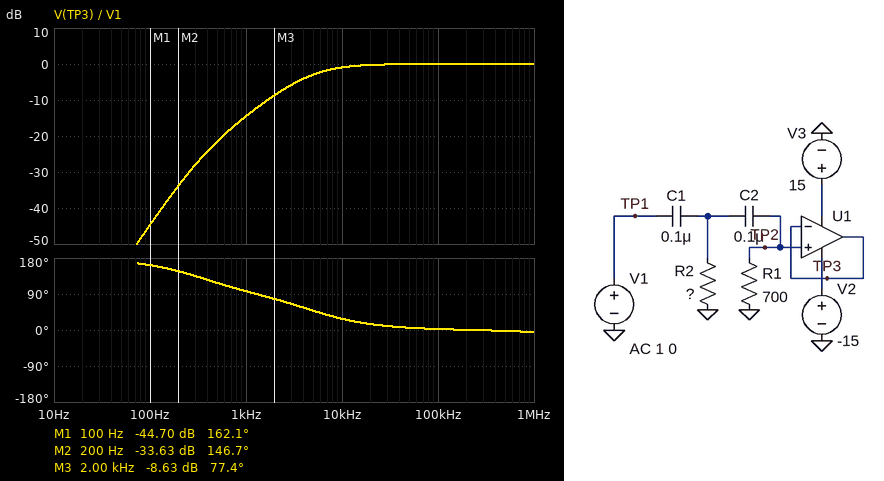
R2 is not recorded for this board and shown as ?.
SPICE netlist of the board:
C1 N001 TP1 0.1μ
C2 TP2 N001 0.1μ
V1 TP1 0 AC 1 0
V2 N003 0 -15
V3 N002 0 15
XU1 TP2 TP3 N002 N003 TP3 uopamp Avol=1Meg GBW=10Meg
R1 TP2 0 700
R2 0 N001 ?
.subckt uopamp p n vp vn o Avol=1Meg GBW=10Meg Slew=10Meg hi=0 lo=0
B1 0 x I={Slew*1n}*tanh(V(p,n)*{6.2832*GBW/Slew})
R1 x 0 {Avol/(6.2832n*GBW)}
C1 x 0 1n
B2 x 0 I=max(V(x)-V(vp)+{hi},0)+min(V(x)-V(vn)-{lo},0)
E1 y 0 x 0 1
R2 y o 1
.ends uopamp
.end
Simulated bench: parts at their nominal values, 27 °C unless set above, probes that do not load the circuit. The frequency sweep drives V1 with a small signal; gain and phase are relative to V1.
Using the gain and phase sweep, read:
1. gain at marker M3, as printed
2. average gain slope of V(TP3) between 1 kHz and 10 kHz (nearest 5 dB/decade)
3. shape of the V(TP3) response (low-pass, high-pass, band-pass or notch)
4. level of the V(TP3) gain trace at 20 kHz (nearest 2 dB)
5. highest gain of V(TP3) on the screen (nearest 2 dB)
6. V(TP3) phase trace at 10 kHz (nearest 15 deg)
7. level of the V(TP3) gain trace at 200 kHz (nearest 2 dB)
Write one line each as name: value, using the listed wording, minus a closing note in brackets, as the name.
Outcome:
gain at marker M3, as printed: -8.63 dB
average gain slope of V(TP3) between 1 kHz and 10 kHz: 15 dB/decade
shape of the V(TP3) response: high-pass
level of the V(TP3) gain trace at 20 kHz: 0 dB
highest gain of V(TP3) on the screen: 0 dB
V(TP3) phase trace at 10 kHz: 30 deg
level of the V(TP3) gain trace at 200 kHz: 0 dB
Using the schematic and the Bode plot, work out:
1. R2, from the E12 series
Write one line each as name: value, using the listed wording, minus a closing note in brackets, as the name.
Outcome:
R2, from the E12 series: 2.2 kΩ
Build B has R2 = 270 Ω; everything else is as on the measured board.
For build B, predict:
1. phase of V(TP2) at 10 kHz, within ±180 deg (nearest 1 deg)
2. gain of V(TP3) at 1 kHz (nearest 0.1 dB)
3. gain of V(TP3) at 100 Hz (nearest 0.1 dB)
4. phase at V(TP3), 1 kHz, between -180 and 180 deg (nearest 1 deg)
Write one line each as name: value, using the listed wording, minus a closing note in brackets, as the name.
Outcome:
phase of V(TP2) at 10 kHz, within ±180 deg: 50 deg
gain of V(TP3) at 1 kHz: -24.2 dB
gain of V(TP3) at 100 Hz: -62.6 dB
phase at V(TP3), 1 kHz, between -180 and 180 deg: 140 deg
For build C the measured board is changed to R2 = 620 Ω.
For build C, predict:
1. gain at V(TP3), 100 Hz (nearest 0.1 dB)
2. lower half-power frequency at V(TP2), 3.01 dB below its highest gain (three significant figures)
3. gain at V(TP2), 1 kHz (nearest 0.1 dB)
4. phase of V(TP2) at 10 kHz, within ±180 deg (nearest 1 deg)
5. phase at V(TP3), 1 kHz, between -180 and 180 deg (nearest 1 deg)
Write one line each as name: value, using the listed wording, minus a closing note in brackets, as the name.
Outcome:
gain at V(TP3), 100 Hz: -55.4 dB
lower half-power frequency at V(TP2), 3.01 dB below its highest gain: 6.31 kHz
gain at V(TP2), 1 kHz: -18.7 dB
phase of V(TP2) at 10 kHz, within ±180 deg: 37 deg
phase at V(TP3), 1 kHz, between -180 and 180 deg: 124 deg
